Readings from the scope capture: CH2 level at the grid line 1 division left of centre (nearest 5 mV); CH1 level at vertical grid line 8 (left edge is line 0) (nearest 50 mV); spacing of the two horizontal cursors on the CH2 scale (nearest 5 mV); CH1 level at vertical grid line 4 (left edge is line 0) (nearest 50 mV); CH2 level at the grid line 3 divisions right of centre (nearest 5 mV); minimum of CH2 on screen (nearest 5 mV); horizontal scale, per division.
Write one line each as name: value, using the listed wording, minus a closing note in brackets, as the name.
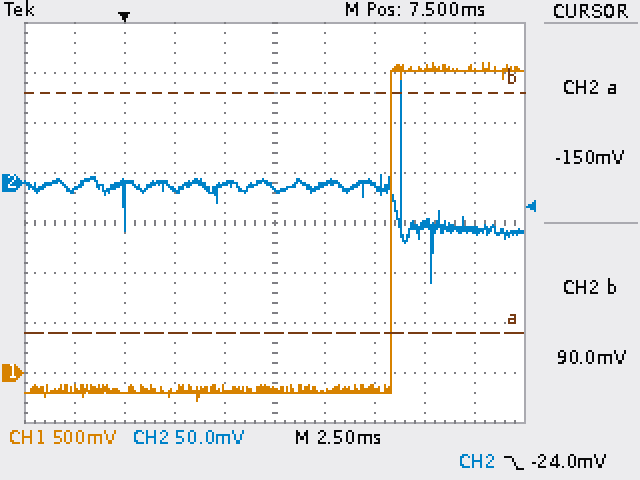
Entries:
CH2 level at the grid line 1 division left of centre: 0 mV
CH1 level at vertical grid line 8 (left edge is line 0): 3.05 V
spacing of the two horizontal cursors on the CH2 scale: 240 mV
CH1 level at vertical grid line 4 (left edge is line 0): -150 mV
CH2 level at the grid line 3 divisions right of centre: -40 mV
minimum of CH2 on screen: -100 mV
horizontal scale, per division: 2.5 ms
